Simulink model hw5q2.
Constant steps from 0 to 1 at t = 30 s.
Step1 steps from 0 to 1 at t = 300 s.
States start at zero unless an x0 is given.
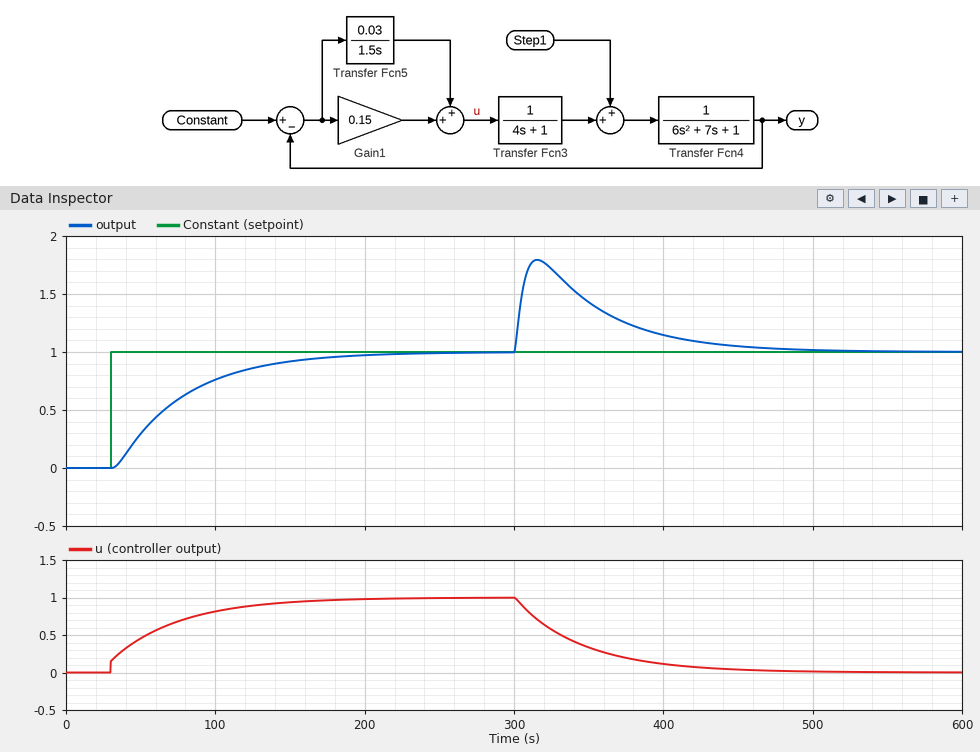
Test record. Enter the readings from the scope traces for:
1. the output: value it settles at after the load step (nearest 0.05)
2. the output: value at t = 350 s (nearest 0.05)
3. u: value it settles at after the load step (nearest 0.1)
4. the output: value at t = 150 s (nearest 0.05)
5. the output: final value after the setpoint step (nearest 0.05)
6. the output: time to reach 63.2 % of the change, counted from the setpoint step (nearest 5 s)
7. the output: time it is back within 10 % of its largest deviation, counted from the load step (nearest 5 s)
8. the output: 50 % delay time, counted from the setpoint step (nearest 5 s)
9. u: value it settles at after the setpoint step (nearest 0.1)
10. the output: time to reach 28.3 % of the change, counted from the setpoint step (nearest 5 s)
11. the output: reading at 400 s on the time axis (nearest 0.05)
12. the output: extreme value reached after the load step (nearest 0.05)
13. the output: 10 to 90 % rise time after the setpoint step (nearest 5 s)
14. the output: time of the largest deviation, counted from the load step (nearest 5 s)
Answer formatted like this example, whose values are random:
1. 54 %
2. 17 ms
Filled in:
1. 1.00
2. 1.45
3. 0.0
4. 0.90
5. 1.00
6. 50 s
7. 130 s
8. 35 s
9. 1.0
10. 20 s
11. 1.15
12. 1.80
13. 100 s
14. 15 s
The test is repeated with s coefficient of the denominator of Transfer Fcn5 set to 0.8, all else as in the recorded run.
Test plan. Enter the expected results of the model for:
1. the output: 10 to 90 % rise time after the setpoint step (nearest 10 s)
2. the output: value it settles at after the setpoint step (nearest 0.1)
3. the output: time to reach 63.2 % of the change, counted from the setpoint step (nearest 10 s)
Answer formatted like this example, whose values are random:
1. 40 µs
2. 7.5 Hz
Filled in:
1. 40 s
2. 1.0
3. 30 s
